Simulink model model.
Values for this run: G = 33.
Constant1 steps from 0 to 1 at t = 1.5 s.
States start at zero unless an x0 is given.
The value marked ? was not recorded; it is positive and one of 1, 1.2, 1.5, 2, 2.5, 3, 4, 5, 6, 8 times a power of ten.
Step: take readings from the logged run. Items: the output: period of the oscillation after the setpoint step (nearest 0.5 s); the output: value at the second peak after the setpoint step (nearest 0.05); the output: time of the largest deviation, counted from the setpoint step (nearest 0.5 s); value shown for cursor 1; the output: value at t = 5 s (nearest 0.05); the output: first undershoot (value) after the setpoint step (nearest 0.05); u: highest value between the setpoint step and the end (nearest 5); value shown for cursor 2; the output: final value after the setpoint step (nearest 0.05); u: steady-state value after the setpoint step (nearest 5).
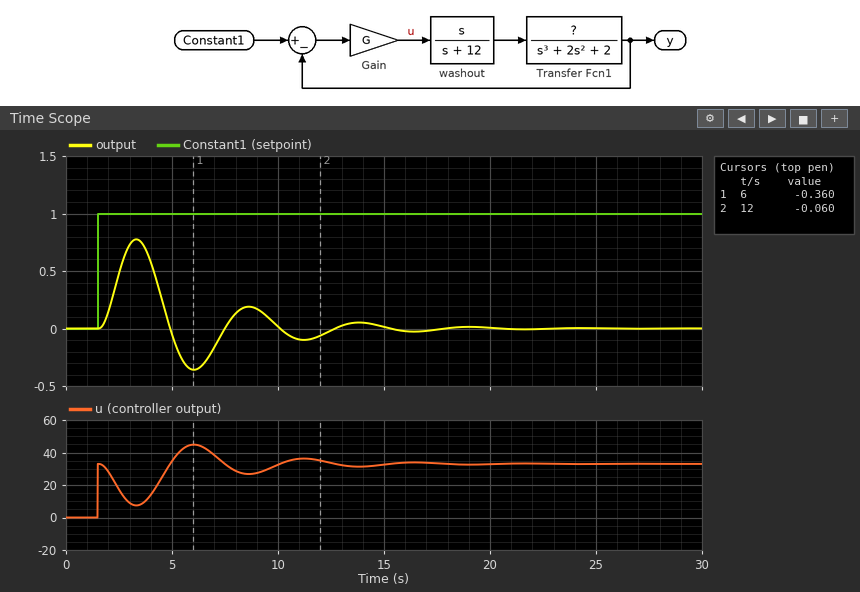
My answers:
5.5 s
0.20
2.0 s
-0.360
-0.05
-0.35
45
-0.060
0.00
35
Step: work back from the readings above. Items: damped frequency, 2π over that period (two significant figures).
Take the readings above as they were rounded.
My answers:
1.1 rad/s
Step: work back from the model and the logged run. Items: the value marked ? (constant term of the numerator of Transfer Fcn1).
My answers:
0.8
